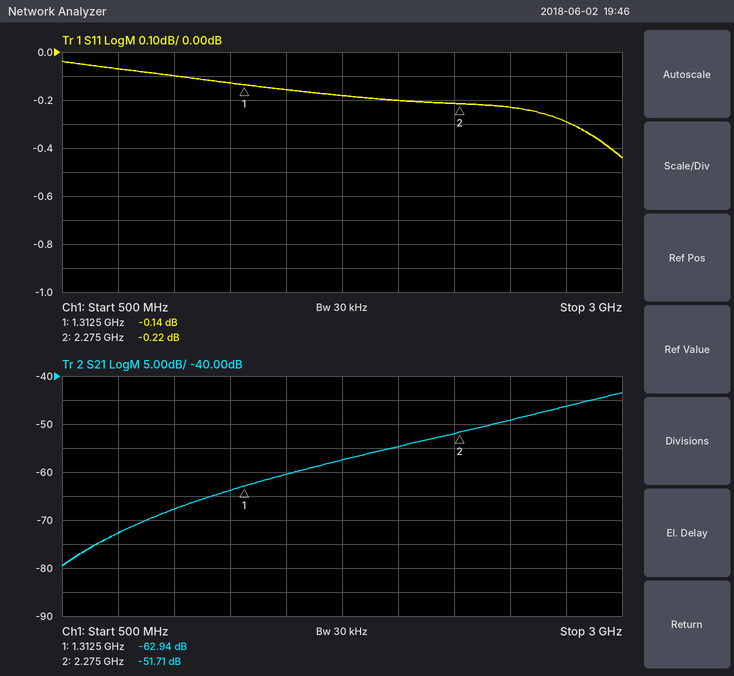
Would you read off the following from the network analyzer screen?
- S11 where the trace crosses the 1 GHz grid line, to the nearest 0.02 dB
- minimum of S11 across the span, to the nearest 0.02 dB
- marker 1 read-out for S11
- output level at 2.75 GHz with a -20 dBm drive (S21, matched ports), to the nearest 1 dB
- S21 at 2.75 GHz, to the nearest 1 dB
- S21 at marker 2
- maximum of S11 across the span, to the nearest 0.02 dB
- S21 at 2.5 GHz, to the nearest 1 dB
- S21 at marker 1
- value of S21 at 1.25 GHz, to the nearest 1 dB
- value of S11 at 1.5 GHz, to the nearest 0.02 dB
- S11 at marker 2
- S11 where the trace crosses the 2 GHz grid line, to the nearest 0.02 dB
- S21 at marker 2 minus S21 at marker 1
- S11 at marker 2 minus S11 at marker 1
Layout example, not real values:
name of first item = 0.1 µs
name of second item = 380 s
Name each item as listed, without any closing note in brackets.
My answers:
S11 where the trace crosses the 1 GHz grid line, to the nearest 0.02 dB = -0.10 dB
minimum of S11 across the span, to the nearest 0.02 dB = -0.44 dB
marker 1 read-out for S11 = -0.14 dB
output level at 2.75 GHz with a -20 dBm drive (S21, matched ports), to the nearest 1 dB = -66 dBm
S21 at 2.75 GHz, to the nearest 1 dB = -46 dB
S21 at marker 2 = -51.71 dB
maximum of S11 across the span, to the nearest 0.02 dB = -0.04 dB
S21 at 2.5 GHz, to the nearest 1 dB = -49 dB
S21 at marker 1 = -62.94 dB
value of S21 at 1.25 GHz, to the nearest 1 dB = -64 dB
value of S11 at 1.5 GHz, to the nearest 0.02 dB = -0.16 dB
S11 at marker 2 = -0.22 dB
S11 where the trace crosses the 2 GHz grid line, to the nearest 0.02 dB = -0.20 dB
S21 at marker 2 minus S21 at marker 1 = 11.23 dB
S11 at marker 2 minus S11 at marker 1 = -0.08 dB
